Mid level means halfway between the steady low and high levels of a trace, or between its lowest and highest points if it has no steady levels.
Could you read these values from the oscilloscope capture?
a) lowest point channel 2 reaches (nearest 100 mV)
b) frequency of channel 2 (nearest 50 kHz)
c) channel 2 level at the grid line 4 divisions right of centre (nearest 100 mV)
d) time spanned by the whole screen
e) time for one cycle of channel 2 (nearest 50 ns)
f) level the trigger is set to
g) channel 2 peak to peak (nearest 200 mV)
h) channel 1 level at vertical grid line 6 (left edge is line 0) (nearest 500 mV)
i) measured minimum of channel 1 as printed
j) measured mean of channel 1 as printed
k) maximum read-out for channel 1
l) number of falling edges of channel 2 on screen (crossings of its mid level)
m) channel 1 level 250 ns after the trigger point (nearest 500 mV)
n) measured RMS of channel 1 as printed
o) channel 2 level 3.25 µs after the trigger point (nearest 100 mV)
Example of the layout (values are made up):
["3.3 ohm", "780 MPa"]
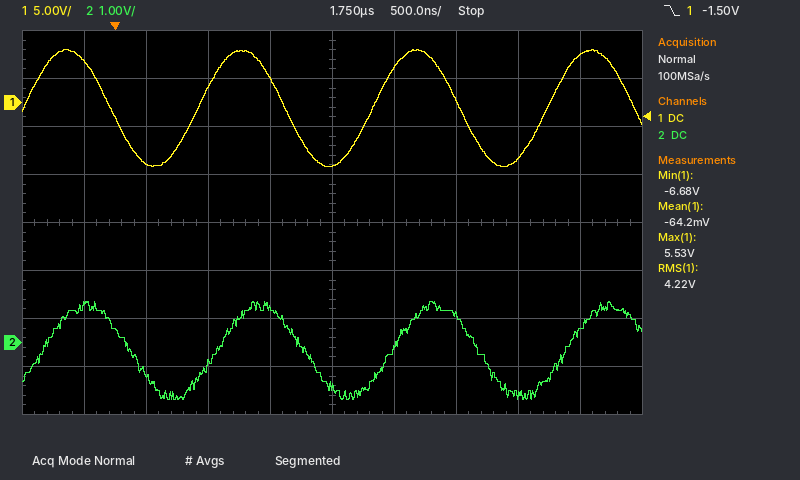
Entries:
["-1.2 V", "700 kHz", "200 mV", "5 µs", "1.40 µs", "-1.50 V", "2.0 V", "3.5 V", "-6.68 V", "-64.2 mV", "5.53 V", "3", "-6.5 V", "4.22 V", "-1.1 V"]
